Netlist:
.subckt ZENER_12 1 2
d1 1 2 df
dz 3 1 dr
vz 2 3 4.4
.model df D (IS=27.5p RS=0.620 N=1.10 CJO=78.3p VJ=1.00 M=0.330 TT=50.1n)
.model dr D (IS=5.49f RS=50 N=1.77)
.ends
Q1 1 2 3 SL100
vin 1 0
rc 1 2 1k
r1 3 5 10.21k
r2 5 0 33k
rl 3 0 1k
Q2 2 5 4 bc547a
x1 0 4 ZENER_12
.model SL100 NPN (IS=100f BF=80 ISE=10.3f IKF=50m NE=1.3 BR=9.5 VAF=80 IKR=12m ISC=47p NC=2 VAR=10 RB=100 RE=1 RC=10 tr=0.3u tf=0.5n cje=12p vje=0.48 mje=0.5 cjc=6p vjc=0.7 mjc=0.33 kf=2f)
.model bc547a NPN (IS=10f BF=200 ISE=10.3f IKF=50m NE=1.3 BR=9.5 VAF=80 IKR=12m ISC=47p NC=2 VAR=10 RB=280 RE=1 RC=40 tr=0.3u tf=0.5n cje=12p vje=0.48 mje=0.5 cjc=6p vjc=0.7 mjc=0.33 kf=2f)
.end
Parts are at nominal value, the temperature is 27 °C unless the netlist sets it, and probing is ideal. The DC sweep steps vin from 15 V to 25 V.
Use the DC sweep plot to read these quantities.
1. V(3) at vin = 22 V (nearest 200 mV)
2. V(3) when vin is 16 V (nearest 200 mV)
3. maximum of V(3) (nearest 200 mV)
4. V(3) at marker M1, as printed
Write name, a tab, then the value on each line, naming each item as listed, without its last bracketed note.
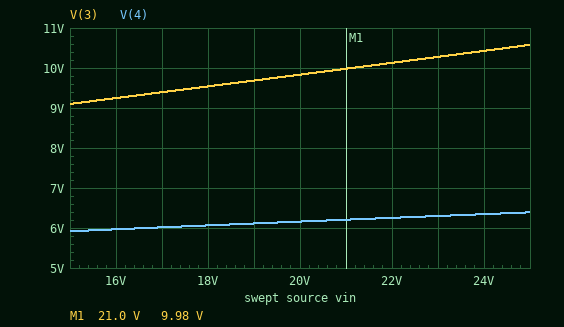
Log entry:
V(3) at vin = 22 V	10.2 V
V(3) when vin is 16 V	9.2 V
maximum of V(3)	10.6 V
V(3) at marker M1, as printed	9.98 V
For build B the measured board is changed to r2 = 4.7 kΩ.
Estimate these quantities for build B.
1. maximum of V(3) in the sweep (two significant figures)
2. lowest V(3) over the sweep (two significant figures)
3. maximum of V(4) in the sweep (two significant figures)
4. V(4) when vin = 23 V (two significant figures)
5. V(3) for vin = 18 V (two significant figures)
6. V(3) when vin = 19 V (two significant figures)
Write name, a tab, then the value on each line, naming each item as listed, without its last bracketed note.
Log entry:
maximum of V(3) in the sweep	21 V
lowest V(3) over the sweep	14 V
maximum of V(4) in the sweep	5.8 V
V(4) when vin = 23 V	5.7 V
V(3) for vin = 18 V	17 V
V(3) when vin = 19 V	18 V
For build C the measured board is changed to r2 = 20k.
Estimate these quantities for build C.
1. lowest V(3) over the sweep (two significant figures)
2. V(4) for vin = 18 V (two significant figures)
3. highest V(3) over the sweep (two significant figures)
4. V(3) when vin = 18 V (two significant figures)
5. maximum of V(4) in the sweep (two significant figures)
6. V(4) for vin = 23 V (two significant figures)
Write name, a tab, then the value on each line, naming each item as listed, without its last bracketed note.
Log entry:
lowest V(3) over the sweep	10 V
V(4) for vin = 18 V	6.0 V
highest V(3) over the sweep	12 V
V(3) when vin = 18 V	11 V
maximum of V(4) in the sweep	6.3 V
V(4) for vin = 23 V	6.2 V
